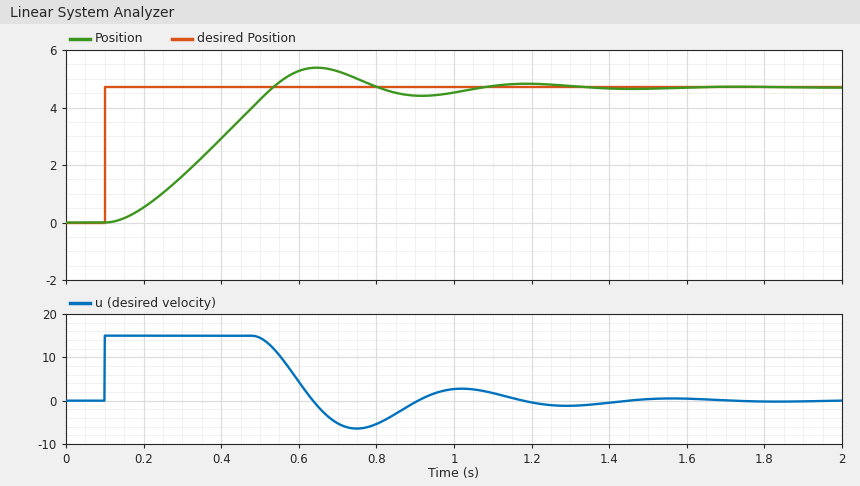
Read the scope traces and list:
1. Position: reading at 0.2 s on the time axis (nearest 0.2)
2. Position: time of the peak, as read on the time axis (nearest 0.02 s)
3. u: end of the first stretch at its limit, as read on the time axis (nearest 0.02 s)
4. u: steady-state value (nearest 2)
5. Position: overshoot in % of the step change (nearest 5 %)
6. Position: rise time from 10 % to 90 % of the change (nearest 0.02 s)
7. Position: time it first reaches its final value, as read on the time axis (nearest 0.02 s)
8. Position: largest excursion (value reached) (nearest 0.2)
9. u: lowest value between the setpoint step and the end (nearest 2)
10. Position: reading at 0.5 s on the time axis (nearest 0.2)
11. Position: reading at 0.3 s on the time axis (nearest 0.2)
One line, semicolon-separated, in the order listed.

0.6; 0.64 s; 0.50 s; 0; 15 %; 0.30 s; 0.54 s; 5.4; -6; 4.2; 1.6
